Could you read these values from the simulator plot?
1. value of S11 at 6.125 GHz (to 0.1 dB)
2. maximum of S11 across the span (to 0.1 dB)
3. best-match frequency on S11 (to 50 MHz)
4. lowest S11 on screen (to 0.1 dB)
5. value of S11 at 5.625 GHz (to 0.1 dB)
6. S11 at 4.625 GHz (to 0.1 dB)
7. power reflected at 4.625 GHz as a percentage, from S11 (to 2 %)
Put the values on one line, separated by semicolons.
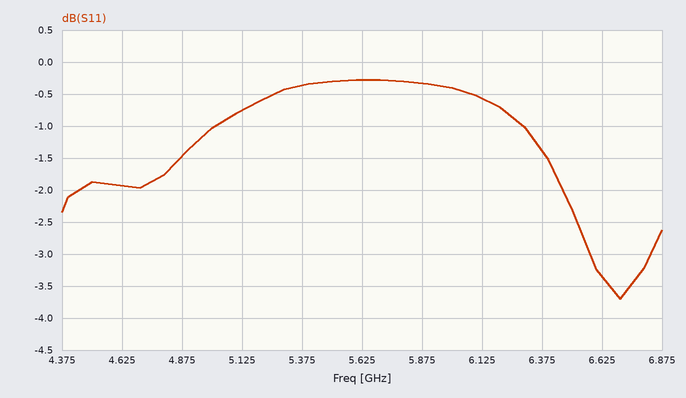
-0.6 dB; -0.3 dB; 6.70 GHz; -3.7 dB; -0.3 dB; -1.9 dB; 64 %
